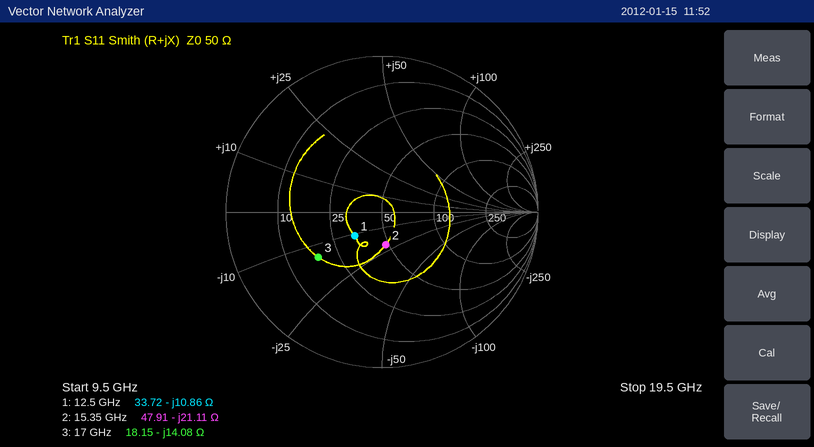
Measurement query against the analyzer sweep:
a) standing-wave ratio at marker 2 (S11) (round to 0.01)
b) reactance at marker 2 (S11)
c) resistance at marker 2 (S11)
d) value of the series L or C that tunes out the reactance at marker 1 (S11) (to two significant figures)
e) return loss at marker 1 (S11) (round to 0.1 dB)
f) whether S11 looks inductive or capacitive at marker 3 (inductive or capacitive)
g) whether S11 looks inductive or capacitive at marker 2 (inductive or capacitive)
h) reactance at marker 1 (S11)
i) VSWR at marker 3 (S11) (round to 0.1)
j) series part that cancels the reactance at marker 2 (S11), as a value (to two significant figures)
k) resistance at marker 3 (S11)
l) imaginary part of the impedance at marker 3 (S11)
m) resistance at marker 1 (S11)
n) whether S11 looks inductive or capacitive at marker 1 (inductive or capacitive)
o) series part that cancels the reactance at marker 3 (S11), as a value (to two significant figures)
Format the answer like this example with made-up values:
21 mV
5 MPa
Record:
1.54
-21.11 Ω
47.91 Ω
140 pH
12.7 dB
capacitive
capacitive
-10.86 Ω
3.0
220 pH
18.15 Ω
-14.08 Ω
33.72 Ω
capacitive
130 pH
